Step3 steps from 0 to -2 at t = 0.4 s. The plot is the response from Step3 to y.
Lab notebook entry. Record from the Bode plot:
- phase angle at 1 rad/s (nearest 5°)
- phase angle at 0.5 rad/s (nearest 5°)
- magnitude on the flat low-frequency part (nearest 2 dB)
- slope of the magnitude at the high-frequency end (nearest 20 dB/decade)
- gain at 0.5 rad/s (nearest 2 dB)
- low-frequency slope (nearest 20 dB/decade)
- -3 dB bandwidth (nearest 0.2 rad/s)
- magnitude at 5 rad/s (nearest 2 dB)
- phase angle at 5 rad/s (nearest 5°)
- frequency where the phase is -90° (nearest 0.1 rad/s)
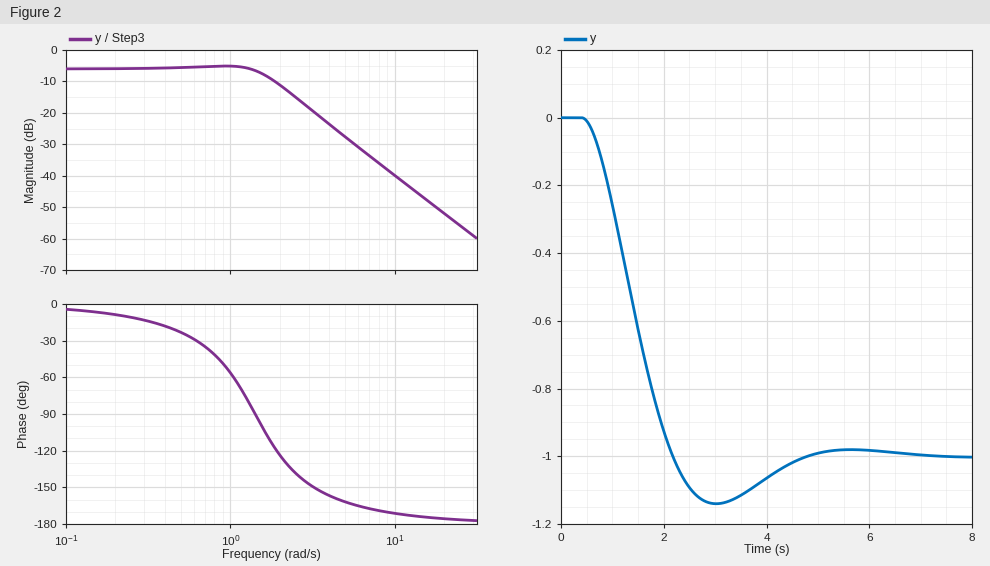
-55°
-25°
-6 dB
-40 dB/decade
-6 dB
0 dB/decade
1.8 rad/s
-28 dB
-160°
1.4 rad/s
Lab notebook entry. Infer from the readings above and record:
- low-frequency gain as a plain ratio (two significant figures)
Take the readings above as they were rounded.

0.50
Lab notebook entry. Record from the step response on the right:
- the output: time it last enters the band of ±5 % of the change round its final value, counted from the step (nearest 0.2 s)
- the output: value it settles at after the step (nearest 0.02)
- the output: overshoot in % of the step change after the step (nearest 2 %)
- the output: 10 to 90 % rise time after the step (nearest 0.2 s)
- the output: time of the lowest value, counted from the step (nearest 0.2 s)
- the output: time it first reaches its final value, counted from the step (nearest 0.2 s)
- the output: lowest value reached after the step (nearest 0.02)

3.8 s
-1.00
14 %
1.2 s
2.6 s
1.8 s
-1.14
